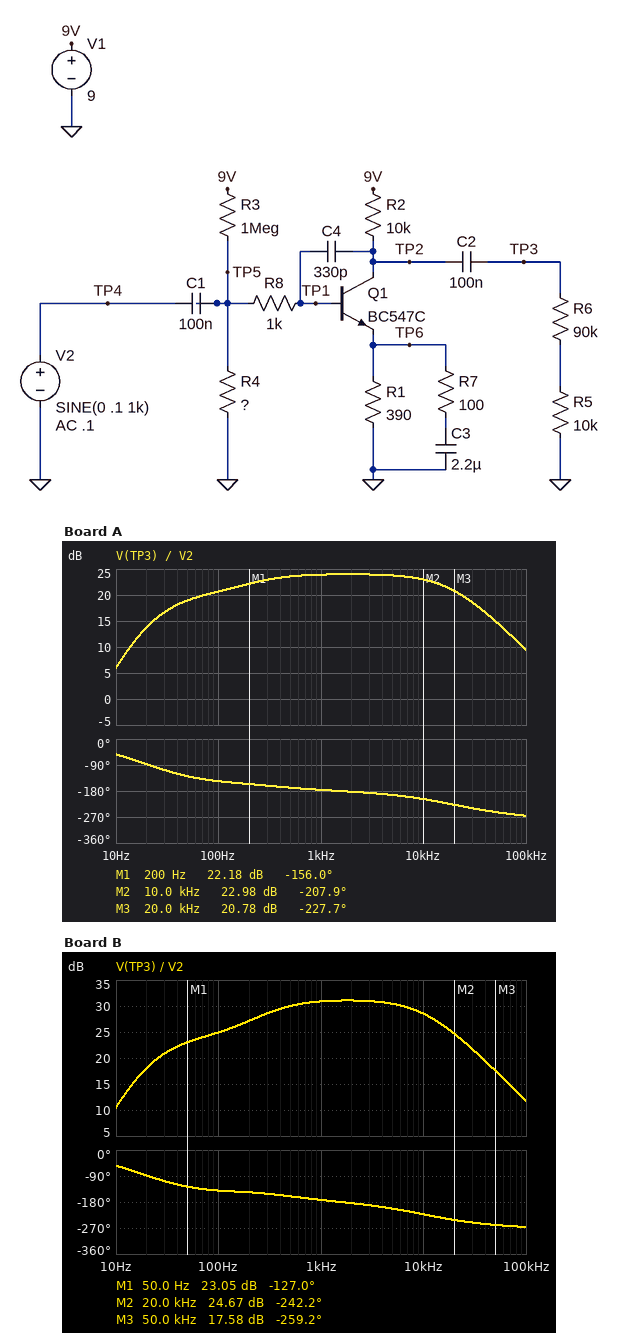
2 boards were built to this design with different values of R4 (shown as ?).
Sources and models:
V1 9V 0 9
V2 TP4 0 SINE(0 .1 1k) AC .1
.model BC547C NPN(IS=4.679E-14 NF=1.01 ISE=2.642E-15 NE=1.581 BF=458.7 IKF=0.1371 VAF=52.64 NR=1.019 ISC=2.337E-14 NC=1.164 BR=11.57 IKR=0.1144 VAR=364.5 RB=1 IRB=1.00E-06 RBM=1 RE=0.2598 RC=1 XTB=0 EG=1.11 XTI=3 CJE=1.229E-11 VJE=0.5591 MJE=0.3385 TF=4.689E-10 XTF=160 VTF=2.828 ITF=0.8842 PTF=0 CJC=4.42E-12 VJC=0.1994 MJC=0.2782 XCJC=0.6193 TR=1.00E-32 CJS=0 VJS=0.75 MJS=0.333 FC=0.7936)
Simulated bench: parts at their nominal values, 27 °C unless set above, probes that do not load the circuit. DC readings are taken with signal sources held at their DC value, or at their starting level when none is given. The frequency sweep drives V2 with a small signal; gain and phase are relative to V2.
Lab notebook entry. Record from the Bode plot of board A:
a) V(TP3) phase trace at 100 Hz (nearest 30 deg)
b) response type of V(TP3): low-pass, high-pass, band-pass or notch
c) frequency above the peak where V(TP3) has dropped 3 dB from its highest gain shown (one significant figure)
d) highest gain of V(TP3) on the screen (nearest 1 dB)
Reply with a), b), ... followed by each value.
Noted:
a) -150 deg
b) band-pass
c) 20 kHz
d) 24 dB
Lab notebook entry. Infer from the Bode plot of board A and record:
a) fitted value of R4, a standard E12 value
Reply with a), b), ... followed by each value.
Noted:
a) 68 kΩ
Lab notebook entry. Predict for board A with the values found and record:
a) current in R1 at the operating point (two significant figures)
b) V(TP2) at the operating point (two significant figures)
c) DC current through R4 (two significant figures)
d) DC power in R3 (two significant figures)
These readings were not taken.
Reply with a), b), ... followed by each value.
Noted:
a) 58 µA
b) 8.4 V
c) 8.3 µA
d) 71 µW
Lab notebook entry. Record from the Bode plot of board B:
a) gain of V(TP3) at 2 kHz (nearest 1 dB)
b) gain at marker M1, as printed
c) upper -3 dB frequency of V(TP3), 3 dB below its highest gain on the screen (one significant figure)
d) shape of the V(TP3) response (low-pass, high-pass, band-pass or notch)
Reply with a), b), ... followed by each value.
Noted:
a) 31 dB
b) 23.05 dB
c) 10 kHz
d) band-pass
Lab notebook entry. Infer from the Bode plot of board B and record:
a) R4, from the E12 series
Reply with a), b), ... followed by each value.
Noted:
a) 82 kΩ
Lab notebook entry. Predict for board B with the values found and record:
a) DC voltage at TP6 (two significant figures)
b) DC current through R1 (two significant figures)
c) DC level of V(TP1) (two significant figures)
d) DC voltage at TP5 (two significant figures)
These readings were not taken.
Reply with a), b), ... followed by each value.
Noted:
a) 77 mV
b) 200 µA
c) 650 mV
d) 650 mV
